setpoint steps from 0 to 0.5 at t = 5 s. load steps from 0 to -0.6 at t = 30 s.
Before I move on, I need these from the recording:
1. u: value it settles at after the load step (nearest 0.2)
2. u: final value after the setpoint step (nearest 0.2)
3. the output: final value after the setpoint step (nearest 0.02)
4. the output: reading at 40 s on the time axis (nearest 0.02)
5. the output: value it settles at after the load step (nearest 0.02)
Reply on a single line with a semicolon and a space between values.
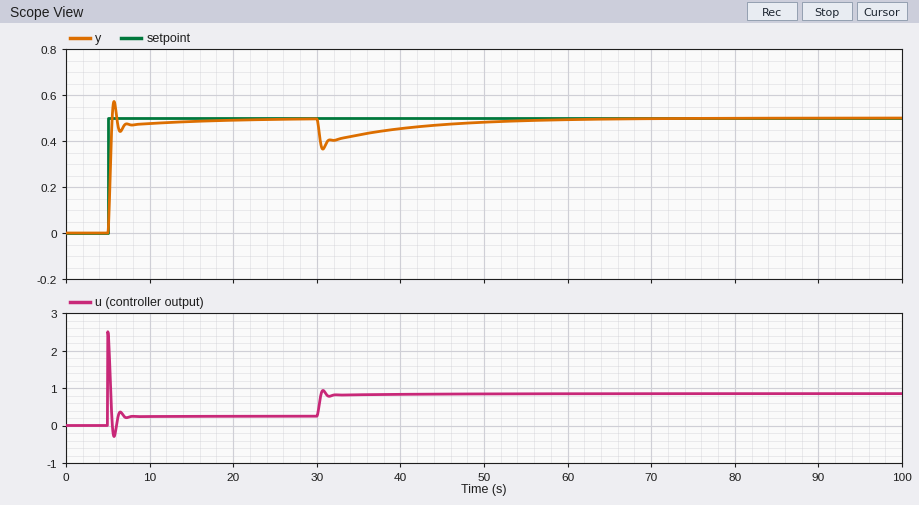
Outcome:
0.8; 0.2; 0.50; 0.46; 0.50
